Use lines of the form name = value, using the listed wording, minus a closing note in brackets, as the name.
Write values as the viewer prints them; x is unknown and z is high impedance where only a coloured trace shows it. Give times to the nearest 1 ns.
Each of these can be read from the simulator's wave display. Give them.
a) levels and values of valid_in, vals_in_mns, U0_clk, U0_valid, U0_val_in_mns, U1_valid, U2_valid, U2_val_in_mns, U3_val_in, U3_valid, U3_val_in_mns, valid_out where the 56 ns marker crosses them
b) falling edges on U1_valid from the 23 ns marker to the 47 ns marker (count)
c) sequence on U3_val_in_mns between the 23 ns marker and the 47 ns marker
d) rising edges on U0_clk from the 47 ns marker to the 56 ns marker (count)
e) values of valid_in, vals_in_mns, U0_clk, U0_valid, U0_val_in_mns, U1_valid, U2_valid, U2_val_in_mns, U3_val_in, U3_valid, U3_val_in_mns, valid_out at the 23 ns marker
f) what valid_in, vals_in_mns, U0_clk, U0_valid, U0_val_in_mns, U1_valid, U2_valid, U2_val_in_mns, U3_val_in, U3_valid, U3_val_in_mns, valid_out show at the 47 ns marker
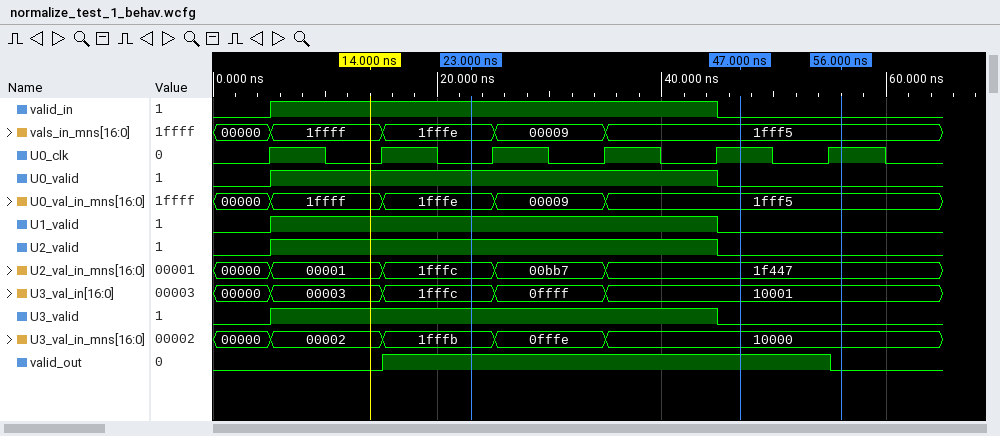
levels and values of valid_in, vals_in_mns, U0_clk, U0_valid, U0_val_in_mns, U1_valid, U2_valid, U2_val_in_mns, U3_val_in, U3_valid, U3_val_in_mns, valid_out where the 56 ns marker crosses them = valid_in=0, vals_in_mns=1fff5, U0_clk=1, U0_valid=0, U0_val_in_mns=1fff5, U1_valid=0, U2_valid=0, U2_val_in_mns=1f447, U3_val_in=10001, U3_valid=0, U3_val_in_mns=10000, valid_out=0
falling edges on U1_valid from the 23 ns marker to the 47 ns marker = 1
sequence on U3_val_in_mns between the 23 ns marker and the 47 ns marker = 1fffb, 0fffe, 10000
rising edges on U0_clk from the 47 ns marker to the 56 ns marker = 1
values of valid_in, vals_in_mns, U0_clk, U0_valid, U0_val_in_mns, U1_valid, U2_valid, U2_val_in_mns, U3_val_in, U3_valid, U3_val_in_mns, valid_out at the 23 ns marker = valid_in=1, vals_in_mns=1fffe, U0_clk=0, U0_valid=1, U0_val_in_mns=1fffe, U1_valid=1, U2_valid=1, U2_val_in_mns=1fffc, U3_val_in=1fffc, U3_valid=1, U3_val_in_mns=1fffb, valid_out=1
what valid_in, vals_in_mns, U0_clk, U0_valid, U0_val_in_mns, U1_valid, U2_valid, U2_val_in_mns, U3_val_in, U3_valid, U3_val_in_mns, valid_out show at the 47 ns marker = valid_in=0, vals_in_mns=1fff5, U0_clk=1, U0_valid=0, U0_val_in_mns=1fff5, U1_valid=0, U2_valid=0, U2_val_in_mns=1f447, U3_val_in=10001, U3_valid=0, U3_val_in_mns=10000, valid_out=1
